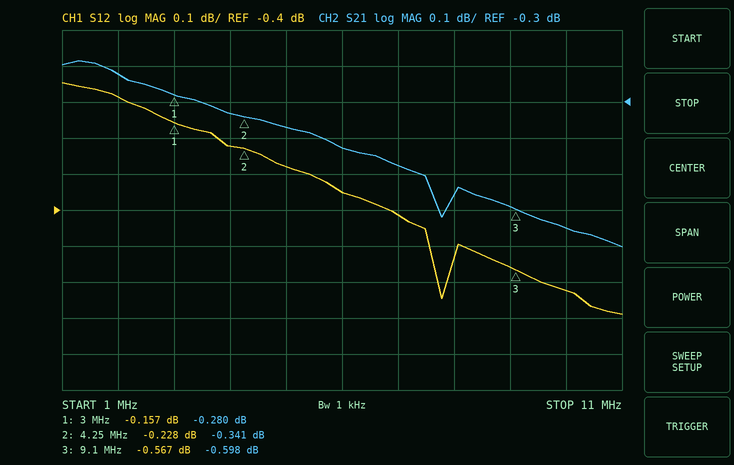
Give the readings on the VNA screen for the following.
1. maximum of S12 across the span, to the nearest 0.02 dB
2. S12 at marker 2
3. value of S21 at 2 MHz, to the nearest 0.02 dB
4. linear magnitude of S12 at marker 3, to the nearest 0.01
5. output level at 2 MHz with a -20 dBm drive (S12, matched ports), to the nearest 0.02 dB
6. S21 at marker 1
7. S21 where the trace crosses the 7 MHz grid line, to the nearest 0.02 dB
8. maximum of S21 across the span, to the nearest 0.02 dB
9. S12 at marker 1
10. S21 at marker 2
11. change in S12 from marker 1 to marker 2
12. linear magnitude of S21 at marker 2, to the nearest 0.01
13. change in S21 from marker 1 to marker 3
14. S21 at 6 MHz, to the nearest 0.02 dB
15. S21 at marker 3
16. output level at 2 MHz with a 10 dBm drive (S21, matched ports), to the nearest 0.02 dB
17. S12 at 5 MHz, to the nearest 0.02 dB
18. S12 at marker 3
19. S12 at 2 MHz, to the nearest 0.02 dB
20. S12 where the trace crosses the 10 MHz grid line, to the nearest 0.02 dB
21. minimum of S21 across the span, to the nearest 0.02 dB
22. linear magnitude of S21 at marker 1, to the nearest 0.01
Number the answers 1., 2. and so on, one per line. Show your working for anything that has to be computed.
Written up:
1. -0.04 dB
2. -0.228 dB
3. -0.22 dB
4. 10^(-0.567/20) ≈ 0.94
5. -20 dBm + (-0.08 dB) = -20.08 dBm
6. -0.280 dB
7. -0.48 dB
8. -0.18 dB
9. -0.157 dB
10. -0.341 dB
11. -0.228 − (-0.157) = -0.071 dB
12. 10^(-0.341/20) ≈ 0.96
13. -0.598 − (-0.28) = -0.318 dB
14. -0.42 dB
15. -0.598 dB
16. 10 dBm + (-0.22 dB) = 9.78 dBm
17. -0.28 dB
18. -0.567 dB
19. -0.08 dB
20. -0.62 dB
21. -0.70 dB
22. 10^(-0.28/20) ≈ 0.97
